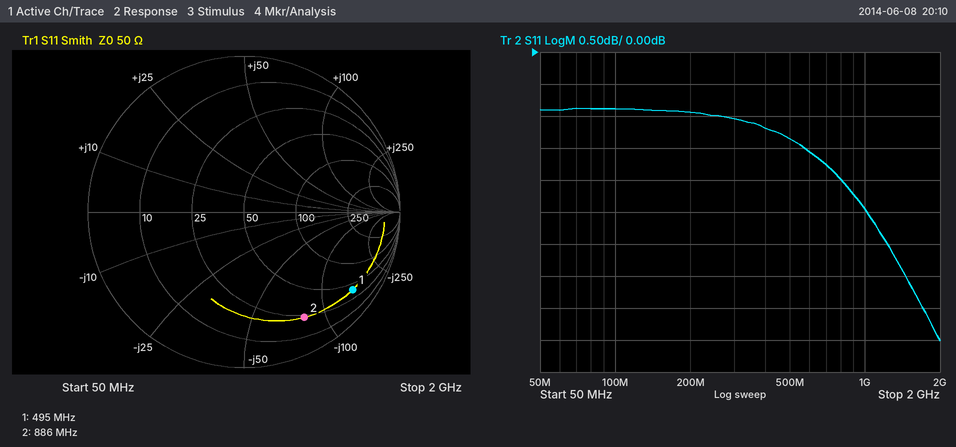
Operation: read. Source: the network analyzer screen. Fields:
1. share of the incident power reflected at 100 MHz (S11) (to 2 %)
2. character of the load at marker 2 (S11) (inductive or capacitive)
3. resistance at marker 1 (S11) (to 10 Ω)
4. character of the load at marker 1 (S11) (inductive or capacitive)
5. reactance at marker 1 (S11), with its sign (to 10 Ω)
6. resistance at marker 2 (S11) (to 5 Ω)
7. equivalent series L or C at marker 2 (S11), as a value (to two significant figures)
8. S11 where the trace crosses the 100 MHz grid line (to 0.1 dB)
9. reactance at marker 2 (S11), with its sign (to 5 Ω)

82 %
capacitive
40 Ω
capacitive
-150 Ω
25 Ω
2.2 pF
-0.9 dB
-80 Ω
